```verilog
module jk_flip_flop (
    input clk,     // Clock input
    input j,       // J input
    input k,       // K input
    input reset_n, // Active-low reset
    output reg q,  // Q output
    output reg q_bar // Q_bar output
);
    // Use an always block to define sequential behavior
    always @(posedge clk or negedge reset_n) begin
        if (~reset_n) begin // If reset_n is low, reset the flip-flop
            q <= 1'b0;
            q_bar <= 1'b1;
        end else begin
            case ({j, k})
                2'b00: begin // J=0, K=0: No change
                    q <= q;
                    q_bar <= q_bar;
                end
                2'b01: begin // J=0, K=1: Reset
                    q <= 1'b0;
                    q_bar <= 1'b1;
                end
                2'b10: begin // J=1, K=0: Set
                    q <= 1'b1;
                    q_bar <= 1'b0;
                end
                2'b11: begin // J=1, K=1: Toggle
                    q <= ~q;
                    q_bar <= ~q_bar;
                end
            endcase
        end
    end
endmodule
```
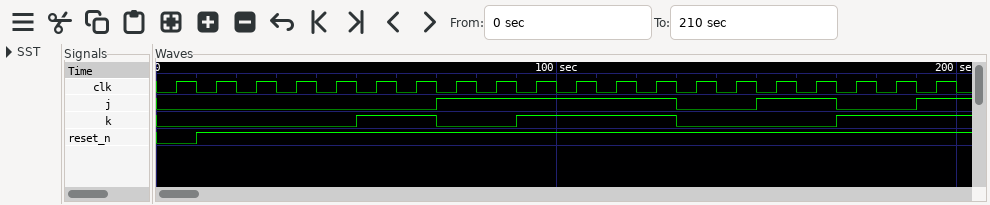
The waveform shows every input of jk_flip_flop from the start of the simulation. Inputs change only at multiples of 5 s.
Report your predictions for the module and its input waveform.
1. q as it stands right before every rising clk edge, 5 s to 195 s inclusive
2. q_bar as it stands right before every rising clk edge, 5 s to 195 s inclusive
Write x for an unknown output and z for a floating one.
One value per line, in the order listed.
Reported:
0 0 0 0 0 0 0 0 1 1 0 1 0 1 1 1 1 1 0 0
1 1 1 1 1 1 1 1 0 0 1 0 1 0 0 0 0 0 1 1
